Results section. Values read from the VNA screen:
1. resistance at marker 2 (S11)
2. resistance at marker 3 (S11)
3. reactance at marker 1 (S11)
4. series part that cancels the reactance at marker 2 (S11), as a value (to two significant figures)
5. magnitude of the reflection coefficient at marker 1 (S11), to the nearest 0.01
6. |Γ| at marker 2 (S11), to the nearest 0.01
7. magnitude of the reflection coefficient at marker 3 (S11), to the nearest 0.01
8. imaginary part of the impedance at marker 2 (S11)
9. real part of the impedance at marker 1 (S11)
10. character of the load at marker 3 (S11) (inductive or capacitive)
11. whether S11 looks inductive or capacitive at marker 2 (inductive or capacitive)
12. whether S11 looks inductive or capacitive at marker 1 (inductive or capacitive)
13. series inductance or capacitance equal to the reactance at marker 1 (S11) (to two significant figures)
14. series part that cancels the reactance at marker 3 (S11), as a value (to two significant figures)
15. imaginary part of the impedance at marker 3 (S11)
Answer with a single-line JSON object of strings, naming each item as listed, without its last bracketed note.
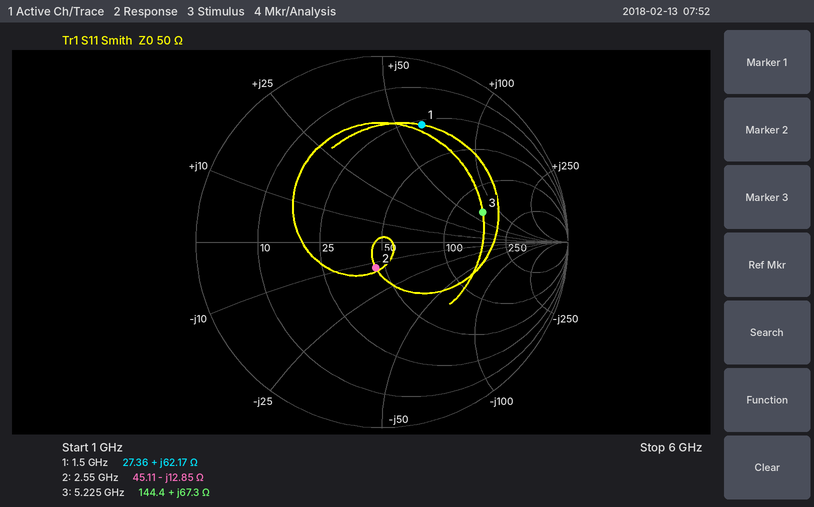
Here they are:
{"resistance at marker 2": "45.11 Ω", "resistance at marker 3": "144.4 Ω", "reactance at marker 1": "+62.17 Ω", "series part that cancels the reactance at marker 2 (S11), as a value": "800 pH", "magnitude of the reflection coefficient at marker 1 (S11), to the nearest 0.01": "0.67", "|Γ| at marker 2 (S11), to the nearest 0.01": "0.14", "magnitude of the reflection coefficient at marker 3 (S11), to the nearest 0.01": "0.56", "imaginary part of the impedance at marker 2": "-12.85 Ω", "real part of the impedance at marker 1": "27.36 Ω", "character of the load at marker 3 (S11)": "inductive", "whether S11 looks inductive or capacitive at marker 2": "capacitive", "whether S11 looks inductive or capacitive at marker 1": "inductive", "series inductance or capacitance equal to the reactance at marker 1 (S11)": "6.6 nH", "series part that cancels the reactance at marker 3 (S11), as a value": "450 fF", "imaginary part of the impedance at marker 3": "+67.3 Ω"}
